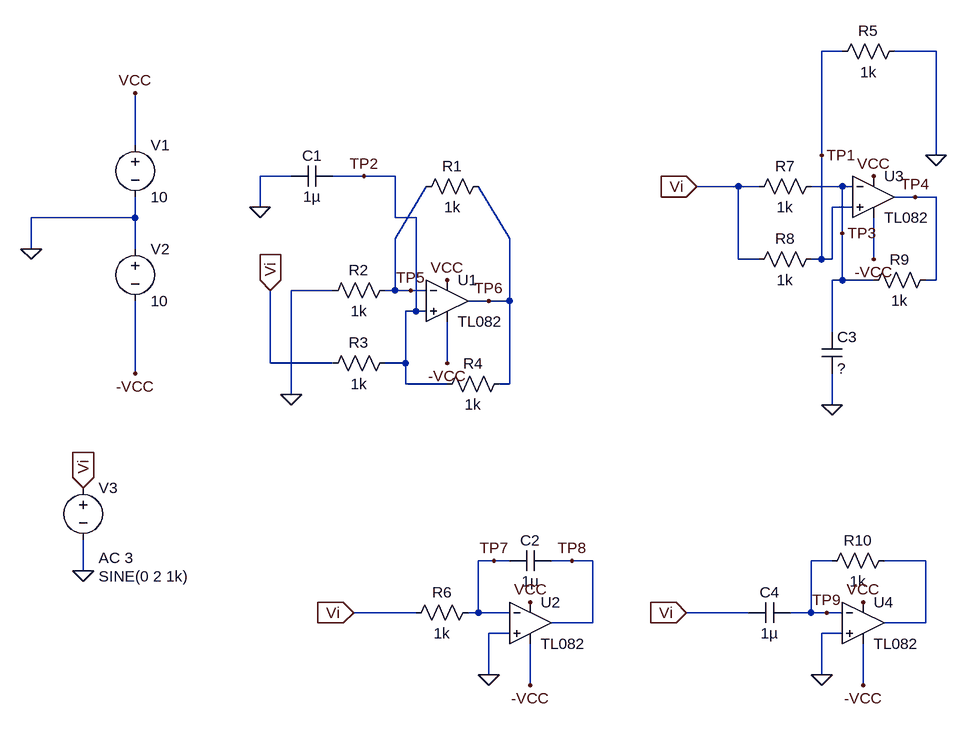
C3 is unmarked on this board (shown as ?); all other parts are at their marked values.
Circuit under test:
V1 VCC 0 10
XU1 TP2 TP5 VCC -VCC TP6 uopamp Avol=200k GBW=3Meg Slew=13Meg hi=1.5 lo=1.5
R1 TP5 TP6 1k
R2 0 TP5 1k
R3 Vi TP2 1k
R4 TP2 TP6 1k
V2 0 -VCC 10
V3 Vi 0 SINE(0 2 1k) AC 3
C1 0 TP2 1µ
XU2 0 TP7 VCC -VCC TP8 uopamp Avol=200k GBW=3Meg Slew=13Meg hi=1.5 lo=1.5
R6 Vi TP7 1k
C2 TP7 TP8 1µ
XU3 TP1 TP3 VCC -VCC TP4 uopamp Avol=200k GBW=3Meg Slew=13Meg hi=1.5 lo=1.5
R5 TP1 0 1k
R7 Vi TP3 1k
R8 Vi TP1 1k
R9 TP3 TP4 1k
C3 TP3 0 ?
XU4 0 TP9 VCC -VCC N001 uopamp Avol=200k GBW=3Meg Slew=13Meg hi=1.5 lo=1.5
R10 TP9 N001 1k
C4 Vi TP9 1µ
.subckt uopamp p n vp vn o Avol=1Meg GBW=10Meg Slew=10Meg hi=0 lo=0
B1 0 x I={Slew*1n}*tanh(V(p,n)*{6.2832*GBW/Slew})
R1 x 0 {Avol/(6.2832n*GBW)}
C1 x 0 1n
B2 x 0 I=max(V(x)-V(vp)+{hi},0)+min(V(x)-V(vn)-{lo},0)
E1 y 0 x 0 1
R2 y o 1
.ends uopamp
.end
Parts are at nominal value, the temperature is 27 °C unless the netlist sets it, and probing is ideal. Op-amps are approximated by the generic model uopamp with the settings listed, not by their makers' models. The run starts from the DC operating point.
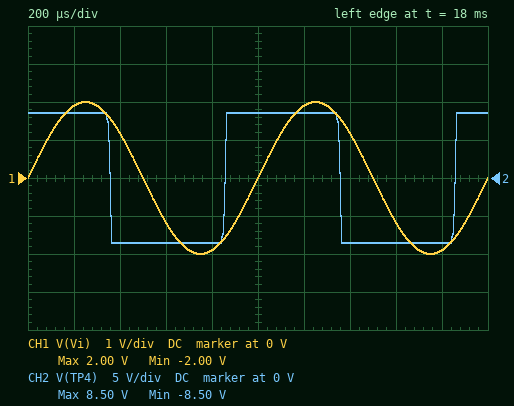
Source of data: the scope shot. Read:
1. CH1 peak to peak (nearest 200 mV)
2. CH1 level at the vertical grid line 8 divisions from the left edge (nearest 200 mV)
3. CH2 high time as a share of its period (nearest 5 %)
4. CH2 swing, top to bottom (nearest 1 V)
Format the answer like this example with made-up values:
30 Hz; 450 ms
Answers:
4.0 V; -1.2 V; 50 %; 17 V
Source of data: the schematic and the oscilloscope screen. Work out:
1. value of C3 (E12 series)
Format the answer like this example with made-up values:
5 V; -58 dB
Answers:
2.7 µF
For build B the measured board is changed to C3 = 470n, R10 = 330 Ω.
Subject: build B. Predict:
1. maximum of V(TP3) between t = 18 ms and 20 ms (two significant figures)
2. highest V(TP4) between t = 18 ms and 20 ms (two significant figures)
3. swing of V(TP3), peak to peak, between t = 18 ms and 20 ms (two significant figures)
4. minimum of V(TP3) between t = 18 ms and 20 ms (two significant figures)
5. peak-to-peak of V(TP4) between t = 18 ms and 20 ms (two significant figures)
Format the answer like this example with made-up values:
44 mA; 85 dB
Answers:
1.0 V; 3.0 V; 2.0 V; -1.0 V; 5.9 V
